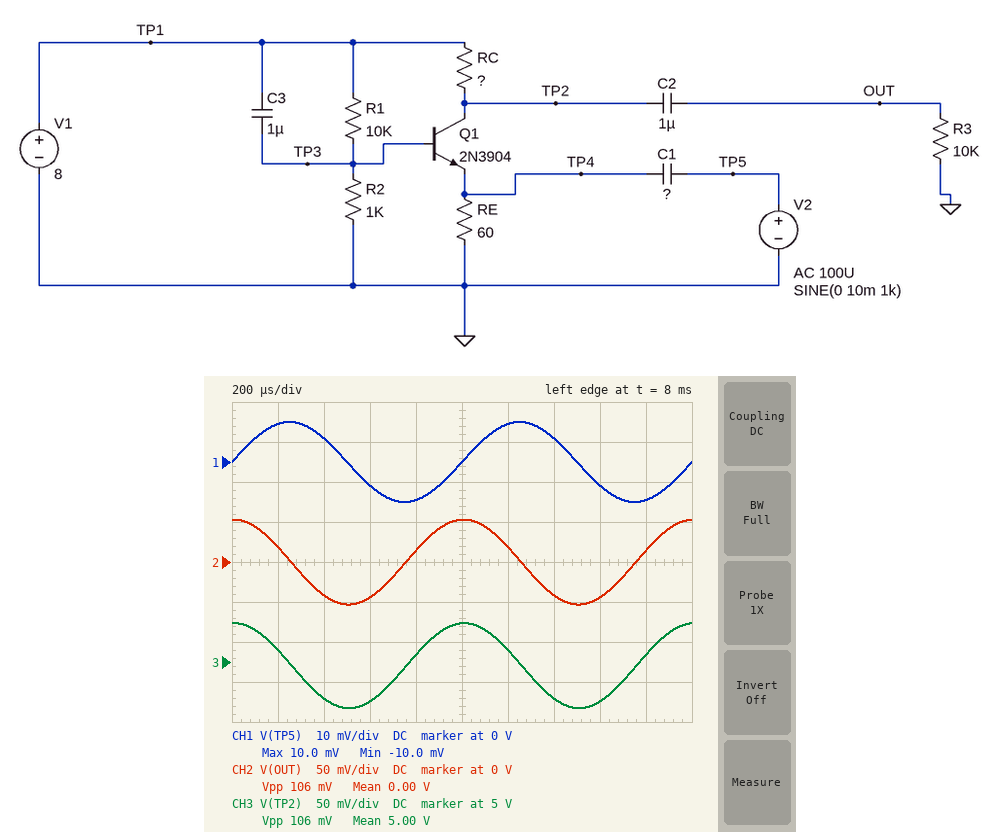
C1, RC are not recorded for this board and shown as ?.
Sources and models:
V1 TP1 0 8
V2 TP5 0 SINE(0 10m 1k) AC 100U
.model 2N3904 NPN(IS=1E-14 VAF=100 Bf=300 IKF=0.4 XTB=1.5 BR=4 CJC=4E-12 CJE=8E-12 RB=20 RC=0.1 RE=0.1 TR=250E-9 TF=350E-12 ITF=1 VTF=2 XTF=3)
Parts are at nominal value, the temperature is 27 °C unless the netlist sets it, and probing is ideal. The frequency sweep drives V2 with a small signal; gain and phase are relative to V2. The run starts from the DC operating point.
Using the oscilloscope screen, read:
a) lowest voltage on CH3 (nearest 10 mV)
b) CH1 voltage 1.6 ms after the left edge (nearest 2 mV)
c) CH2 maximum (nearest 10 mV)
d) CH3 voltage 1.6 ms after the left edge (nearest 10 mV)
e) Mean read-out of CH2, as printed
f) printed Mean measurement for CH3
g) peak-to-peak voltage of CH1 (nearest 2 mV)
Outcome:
4.94 V
-6 mV
50 mV
4.95 V
0.00 V
5.00 V
20 mV
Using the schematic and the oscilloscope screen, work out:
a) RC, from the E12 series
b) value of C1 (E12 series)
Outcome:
2.7 kΩ
560 nF
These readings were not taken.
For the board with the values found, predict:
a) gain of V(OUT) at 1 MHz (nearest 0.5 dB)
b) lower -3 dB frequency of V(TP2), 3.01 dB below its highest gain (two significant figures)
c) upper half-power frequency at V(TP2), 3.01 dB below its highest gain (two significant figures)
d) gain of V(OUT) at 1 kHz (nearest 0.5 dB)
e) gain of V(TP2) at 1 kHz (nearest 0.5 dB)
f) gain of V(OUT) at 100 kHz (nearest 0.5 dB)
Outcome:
39.0 dB
17 kHz
19 MHz
14.5 dB
14.5 dB
39.0 dB
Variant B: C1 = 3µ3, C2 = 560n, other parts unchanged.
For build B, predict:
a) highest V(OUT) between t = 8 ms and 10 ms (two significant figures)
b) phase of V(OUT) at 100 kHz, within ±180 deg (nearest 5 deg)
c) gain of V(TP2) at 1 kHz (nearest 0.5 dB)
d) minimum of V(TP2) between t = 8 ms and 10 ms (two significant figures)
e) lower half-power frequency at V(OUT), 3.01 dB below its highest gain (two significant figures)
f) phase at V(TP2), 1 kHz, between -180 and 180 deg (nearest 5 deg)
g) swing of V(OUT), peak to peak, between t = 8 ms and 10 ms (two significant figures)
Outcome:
290 mV
0 deg
29.5 dB
4.7 V
2.8 kHz
70 deg
590 mV
